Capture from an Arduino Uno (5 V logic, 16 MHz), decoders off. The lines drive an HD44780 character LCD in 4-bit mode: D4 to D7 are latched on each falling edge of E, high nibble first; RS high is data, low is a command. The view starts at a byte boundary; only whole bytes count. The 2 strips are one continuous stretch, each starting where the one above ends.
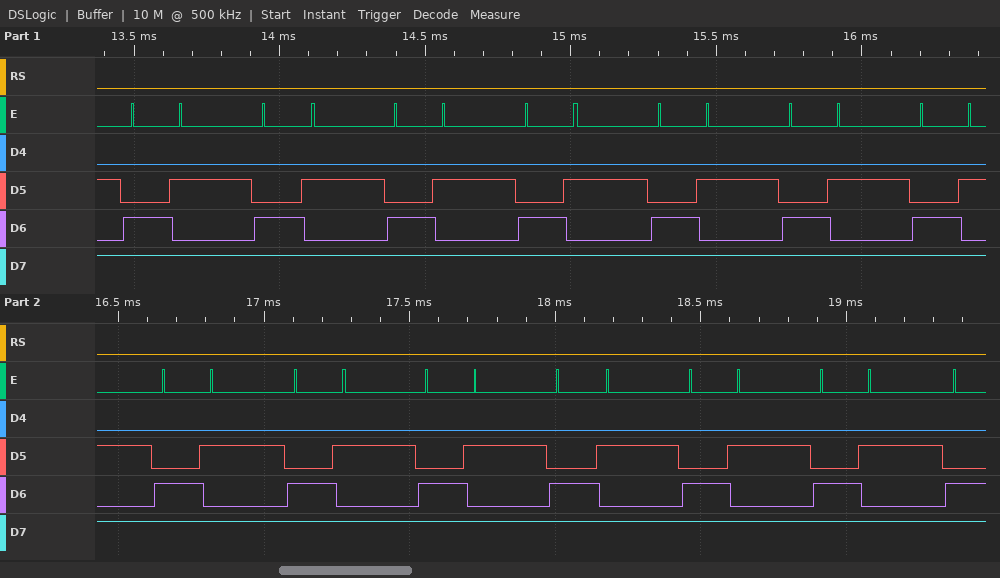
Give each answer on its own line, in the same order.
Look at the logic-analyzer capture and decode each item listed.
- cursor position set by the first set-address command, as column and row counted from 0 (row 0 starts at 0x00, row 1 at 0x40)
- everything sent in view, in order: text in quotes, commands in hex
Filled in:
column 10, row 1
0xCA 0xCA 0xCA 0xCA 0xCA 0xCA 0xCA 0xCA 0xCA 0xCA 0xCA 0xCA 0xCA
